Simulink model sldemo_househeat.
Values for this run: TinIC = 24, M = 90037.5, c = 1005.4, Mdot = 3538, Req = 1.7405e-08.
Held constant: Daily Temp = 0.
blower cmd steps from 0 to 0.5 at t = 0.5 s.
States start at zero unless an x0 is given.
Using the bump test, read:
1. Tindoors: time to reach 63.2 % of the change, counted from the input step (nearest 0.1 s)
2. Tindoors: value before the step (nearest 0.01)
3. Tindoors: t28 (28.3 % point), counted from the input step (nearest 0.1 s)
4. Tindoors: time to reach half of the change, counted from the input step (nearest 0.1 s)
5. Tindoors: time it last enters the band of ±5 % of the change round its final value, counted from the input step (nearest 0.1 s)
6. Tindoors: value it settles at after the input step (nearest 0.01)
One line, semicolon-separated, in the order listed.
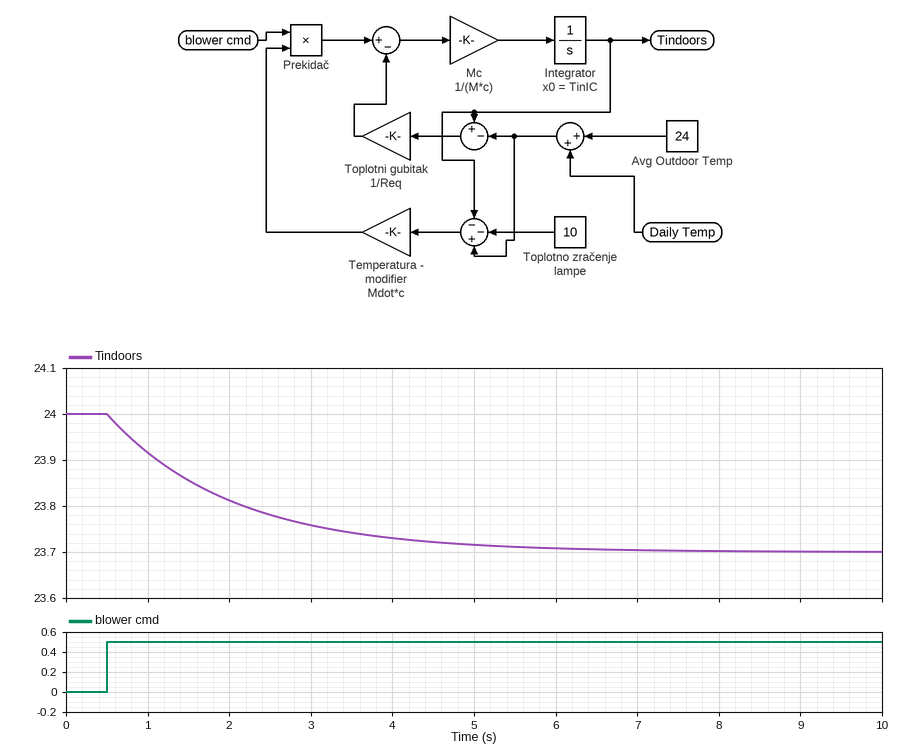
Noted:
1.5 s; 24.00; 0.5 s; 1.1 s; 4.6 s; 23.70
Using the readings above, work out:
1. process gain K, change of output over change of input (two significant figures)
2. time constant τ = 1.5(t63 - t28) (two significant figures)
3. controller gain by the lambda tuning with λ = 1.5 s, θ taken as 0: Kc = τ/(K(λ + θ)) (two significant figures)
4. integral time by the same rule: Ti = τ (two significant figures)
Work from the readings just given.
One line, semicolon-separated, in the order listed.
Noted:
-0.60; 1.5 s; -1.7; 1.5 s
